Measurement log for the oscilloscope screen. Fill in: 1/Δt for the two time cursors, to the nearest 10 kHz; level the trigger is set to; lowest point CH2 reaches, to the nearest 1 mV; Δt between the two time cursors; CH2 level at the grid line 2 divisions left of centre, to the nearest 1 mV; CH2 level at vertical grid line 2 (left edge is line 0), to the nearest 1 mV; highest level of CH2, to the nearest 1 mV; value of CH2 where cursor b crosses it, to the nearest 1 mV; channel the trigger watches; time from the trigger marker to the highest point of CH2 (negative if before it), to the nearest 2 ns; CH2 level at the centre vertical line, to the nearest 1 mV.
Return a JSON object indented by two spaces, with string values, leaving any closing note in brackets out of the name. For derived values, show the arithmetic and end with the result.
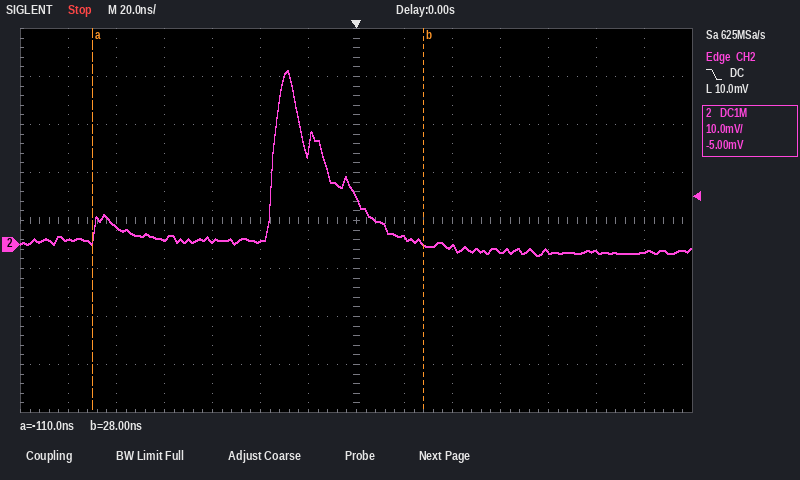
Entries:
{
  "1/Δt for the two time cursors, to the nearest 10 kHz": "1 / 138 ns ≈ 7.25 MHz",
  "level the trigger is set to": "10.0 mV",
  "lowest point CH2 reaches, to the nearest 1 mV": "-2 mV",
  "Δt between the two time cursors": "28 ns − (-110 ns) = 138 ns",
  "CH2 level at the grid line 2 divisions left of centre, to the nearest 1 mV": "1 mV",
  "CH2 level at vertical grid line 2 (left edge is line 0), to the nearest 1 mV": "4 mV",
  "highest level of CH2, to the nearest 1 mV": "36 mV",
  "value of CH2 where cursor b crosses it, to the nearest 1 mV": "0 mV",
  "channel the trigger watches": "CH2",
  "time from the trigger marker to the highest point of CH2 (negative if before it), to the nearest 2 ns": "-28 ns",
  "CH2 level at the centre vertical line, to the nearest 1 mV": "10 mV"
}
